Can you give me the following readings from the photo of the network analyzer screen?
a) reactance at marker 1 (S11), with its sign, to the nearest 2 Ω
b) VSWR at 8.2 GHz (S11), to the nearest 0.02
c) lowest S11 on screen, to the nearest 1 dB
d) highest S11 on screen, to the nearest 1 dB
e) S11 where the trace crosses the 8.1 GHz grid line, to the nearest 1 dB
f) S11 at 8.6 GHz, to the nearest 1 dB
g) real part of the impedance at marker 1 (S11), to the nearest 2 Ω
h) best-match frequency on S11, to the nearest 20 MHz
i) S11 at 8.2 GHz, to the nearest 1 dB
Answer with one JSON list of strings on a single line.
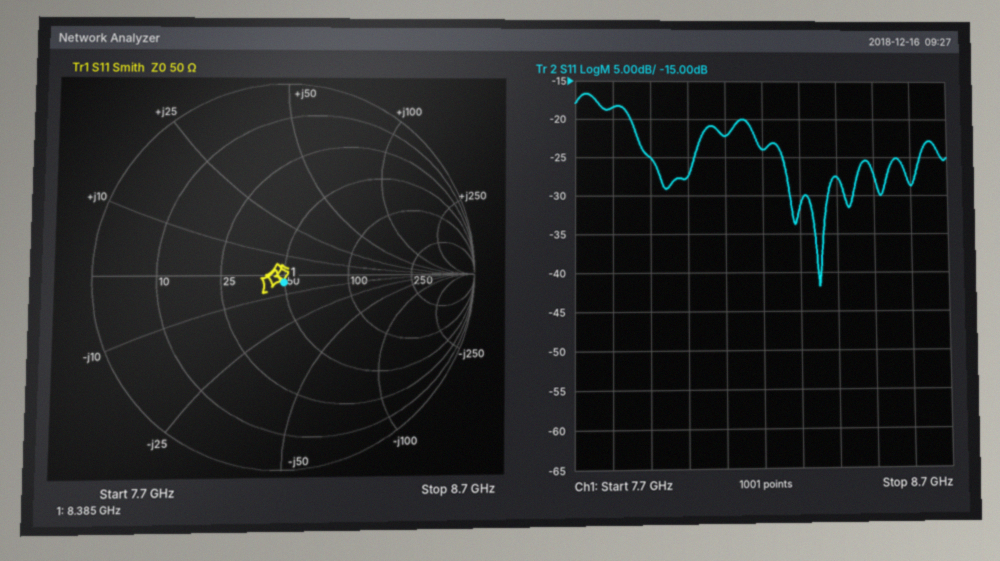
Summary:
["-4 Ω", "1.14", "-42 dB", "-17 dB", "-22 dB", "-29 dB", "50 Ω", "8.36 GHz", "-24 dB"]
